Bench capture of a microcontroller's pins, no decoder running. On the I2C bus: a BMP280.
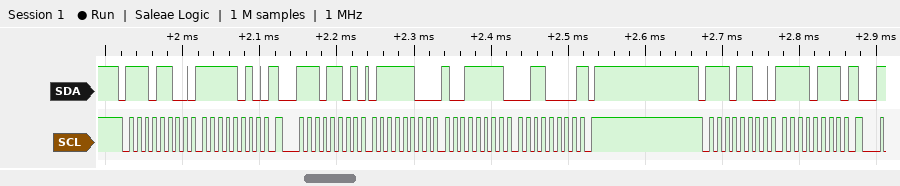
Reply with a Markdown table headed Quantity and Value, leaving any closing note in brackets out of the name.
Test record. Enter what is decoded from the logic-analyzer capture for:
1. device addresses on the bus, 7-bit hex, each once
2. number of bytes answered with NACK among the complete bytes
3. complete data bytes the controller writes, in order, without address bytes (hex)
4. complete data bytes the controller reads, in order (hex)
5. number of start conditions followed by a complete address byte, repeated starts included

| Quantity | Value |
|---|---|
| device addresses on the bus, 7-bit hex, each once | 0x76 |
| number of bytes answered with NACK among the complete bytes | 1 |
| complete data bytes the controller writes, in order, without address bytes | FA F7 |
| complete data bytes the controller reads, in order | 7C 9F 30 |
| number of start conditions followed by a complete address byte, repeated starts included | 3 |
